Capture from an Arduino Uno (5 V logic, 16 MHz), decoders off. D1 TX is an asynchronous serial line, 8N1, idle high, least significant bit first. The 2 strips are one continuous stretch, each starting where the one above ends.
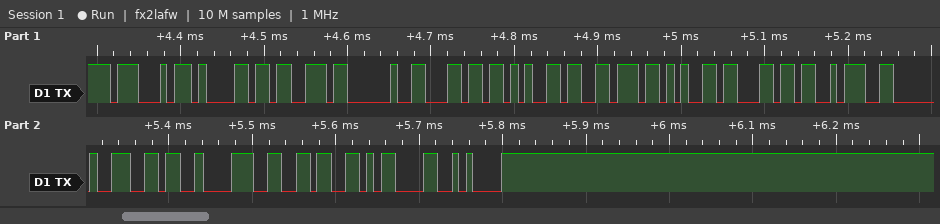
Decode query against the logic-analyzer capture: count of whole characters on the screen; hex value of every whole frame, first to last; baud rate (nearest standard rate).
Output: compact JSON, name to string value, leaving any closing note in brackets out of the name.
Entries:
{"count of whole characters on the screen": "16", "hex value of every whole frame, first to last": "0x47 0x61 0x73 0x20 0x6C 0x65 0x76 0x65 0x6C 0x3A 0x20 0x36 0x38 0x36 0x0D 0x0A", "baud rate": "115200 baud"}
